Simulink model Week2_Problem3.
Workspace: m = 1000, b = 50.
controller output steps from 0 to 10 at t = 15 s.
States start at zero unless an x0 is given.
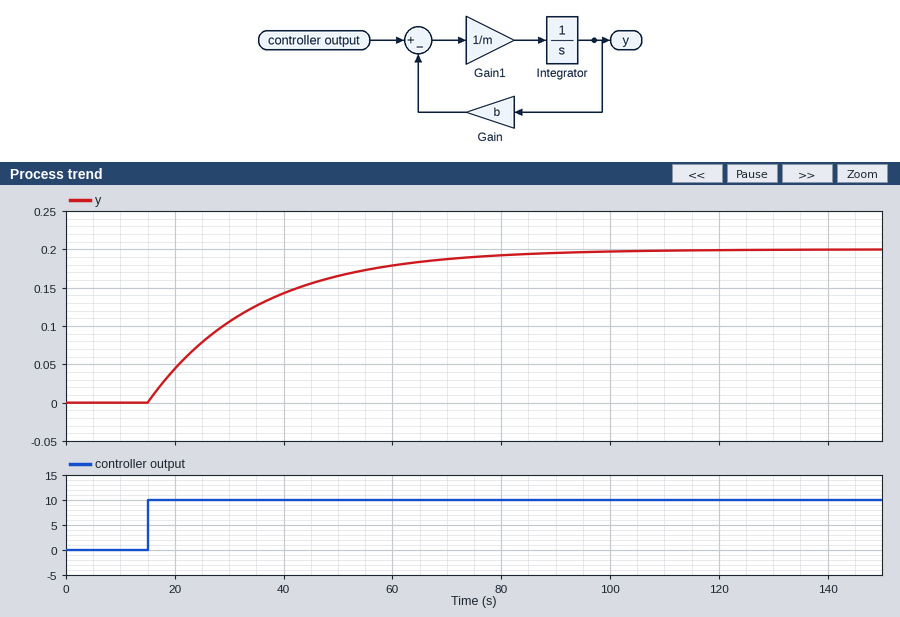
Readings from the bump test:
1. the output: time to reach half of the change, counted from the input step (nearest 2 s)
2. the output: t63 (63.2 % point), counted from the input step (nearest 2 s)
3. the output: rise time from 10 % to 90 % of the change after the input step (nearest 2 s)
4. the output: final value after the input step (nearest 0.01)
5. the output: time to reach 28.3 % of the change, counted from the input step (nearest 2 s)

14 s
20 s
44 s
0.20
6 s
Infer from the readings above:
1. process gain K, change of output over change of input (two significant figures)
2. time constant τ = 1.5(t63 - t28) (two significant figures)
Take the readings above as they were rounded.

0.020
21 s
